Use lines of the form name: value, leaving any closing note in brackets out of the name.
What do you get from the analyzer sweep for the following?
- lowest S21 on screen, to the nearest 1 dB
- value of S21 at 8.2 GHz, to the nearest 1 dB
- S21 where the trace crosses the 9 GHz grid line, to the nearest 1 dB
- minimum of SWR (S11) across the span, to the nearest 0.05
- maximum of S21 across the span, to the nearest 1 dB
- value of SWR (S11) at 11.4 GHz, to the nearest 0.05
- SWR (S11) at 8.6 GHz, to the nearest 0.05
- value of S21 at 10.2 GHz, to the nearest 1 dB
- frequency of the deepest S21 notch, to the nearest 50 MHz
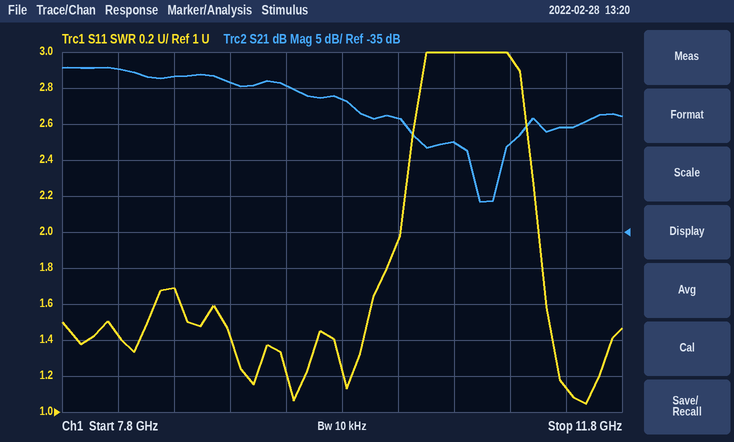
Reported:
lowest S21 on screen, to the nearest 1 dB: -31 dB
value of S21 at 8.2 GHz, to the nearest 1 dB: -12 dB
S21 where the trace crosses the 9 GHz grid line, to the nearest 1 dB: -14 dB
minimum of SWR (S11) across the span, to the nearest 0.05: 1.05
maximum of S21 across the span, to the nearest 1 dB: -12 dB
value of SWR (S11) at 11.4 GHz, to the nearest 0.05: 1.15
SWR (S11) at 8.6 GHz, to the nearest 0.05: 1.70
value of S21 at 10.2 GHz, to the nearest 1 dB: -19 dB
frequency of the deepest S21 notch, to the nearest 50 MHz: 10.80 GHz
